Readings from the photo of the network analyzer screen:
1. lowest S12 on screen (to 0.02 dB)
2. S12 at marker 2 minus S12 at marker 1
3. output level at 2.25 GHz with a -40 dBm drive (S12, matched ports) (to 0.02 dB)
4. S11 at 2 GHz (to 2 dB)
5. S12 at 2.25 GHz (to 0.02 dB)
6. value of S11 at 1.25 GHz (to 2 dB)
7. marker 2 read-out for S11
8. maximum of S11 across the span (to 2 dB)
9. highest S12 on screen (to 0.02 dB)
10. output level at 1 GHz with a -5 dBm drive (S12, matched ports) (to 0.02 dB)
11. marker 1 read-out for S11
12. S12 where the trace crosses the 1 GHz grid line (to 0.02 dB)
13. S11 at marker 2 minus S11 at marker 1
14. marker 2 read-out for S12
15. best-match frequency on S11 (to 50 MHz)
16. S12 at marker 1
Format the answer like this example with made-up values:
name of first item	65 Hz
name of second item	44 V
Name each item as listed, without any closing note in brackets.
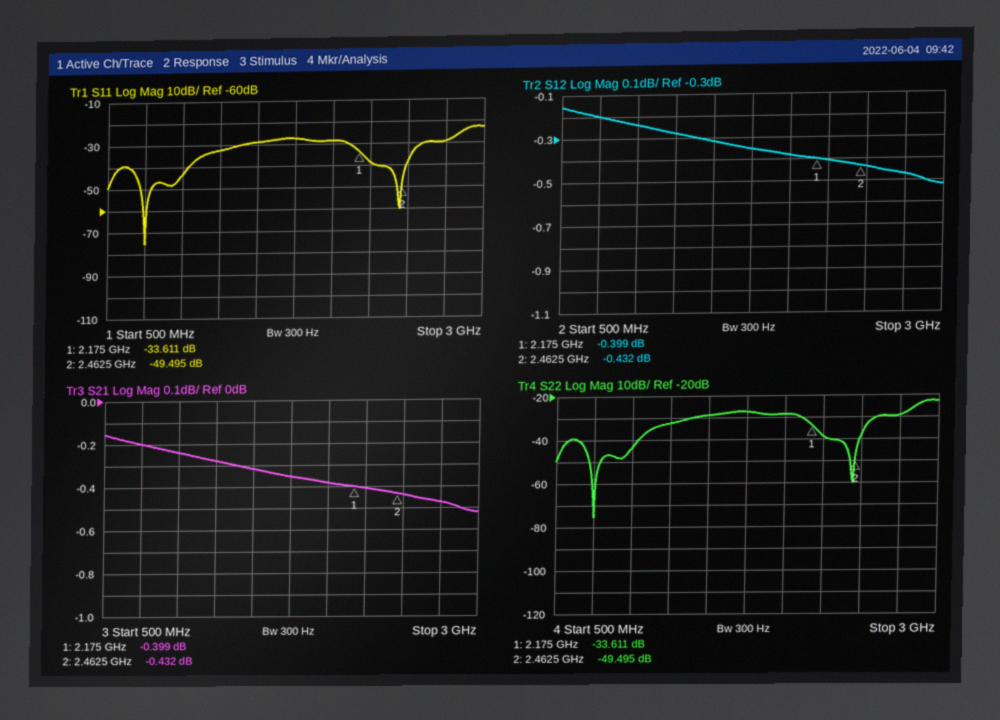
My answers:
lowest S12 on screen	-0.52 dB
S12 at marker 2 minus S12 at marker 1	-0.033 dB
output level at 2.25 GHz with a -40 dBm drive (S12, matched ports)	-40.40 dBm
S11 at 2 GHz	-28 dB
S12 at 2.25 GHz	-0.40 dB
value of S11 at 1.25 GHz	-32 dB
marker 2 read-out for S11	-49.495 dB
maximum of S11 across the span	-22 dB
highest S12 on screen	-0.16 dB
output level at 1 GHz with a -5 dBm drive (S12, matched ports)	-5.24 dBm
marker 1 read-out for S11	-33.611 dB
S12 where the trace crosses the 1 GHz grid line	-0.24 dB
S11 at marker 2 minus S11 at marker 1	-15.884 dB
marker 2 read-out for S12	-0.432 dB
best-match frequency on S11	750 MHz
S12 at marker 1	-0.399 dB
